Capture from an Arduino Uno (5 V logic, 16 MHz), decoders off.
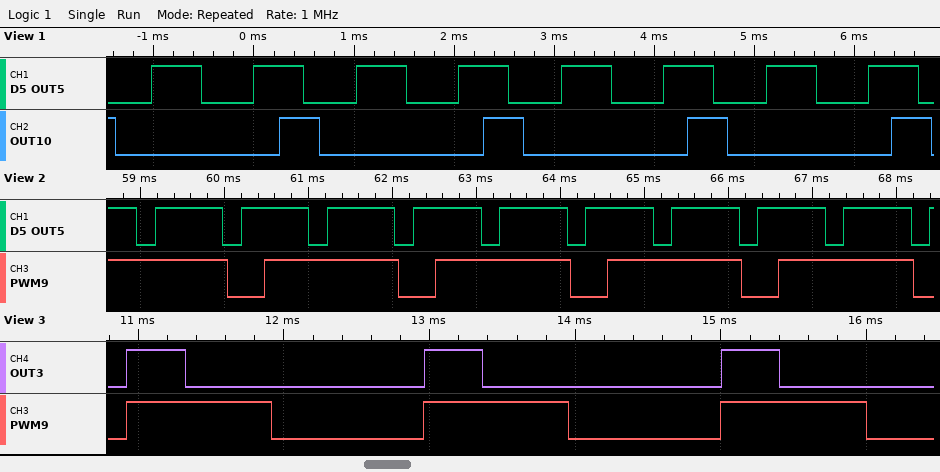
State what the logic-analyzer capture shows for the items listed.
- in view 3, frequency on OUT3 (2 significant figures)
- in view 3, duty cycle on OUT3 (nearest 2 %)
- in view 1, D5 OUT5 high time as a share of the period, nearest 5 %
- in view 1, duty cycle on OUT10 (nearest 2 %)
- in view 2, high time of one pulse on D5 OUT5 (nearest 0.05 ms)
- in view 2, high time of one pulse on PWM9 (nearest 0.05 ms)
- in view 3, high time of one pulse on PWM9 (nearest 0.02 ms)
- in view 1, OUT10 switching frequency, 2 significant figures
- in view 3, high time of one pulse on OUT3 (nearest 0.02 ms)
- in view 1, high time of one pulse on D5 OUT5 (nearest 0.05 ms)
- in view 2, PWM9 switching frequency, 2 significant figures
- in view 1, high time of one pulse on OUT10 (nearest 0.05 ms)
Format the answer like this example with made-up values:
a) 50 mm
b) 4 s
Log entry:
a) 490 Hz
b) 20 %
c) 50 %
d) 20 %
e) 0.80 ms
f) 1.60 ms
g) 1.00 ms
h) 490 Hz
i) 0.40 ms
j) 0.50 ms
k) 490 Hz
l) 0.40 ms
